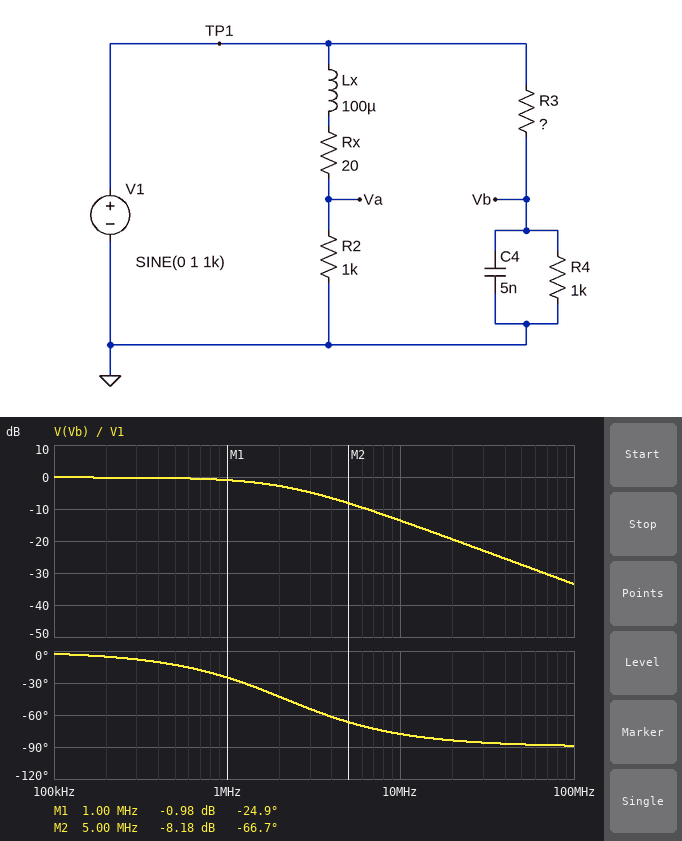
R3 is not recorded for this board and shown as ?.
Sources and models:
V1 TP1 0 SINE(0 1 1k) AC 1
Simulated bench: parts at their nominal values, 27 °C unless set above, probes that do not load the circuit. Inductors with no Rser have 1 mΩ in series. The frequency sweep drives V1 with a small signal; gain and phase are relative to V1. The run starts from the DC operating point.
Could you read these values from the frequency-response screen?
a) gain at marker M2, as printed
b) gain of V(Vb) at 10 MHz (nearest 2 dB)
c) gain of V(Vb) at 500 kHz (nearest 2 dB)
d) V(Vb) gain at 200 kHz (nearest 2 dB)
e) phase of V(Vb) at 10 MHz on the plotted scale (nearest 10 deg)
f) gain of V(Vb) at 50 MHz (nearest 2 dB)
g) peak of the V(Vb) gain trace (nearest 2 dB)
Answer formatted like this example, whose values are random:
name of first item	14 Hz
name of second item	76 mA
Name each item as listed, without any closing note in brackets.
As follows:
gain at marker M2, as printed	-8.18 dB
gain of V(Vb) at 10 MHz	-14 dB
gain of V(Vb) at 500 kHz	0 dB
V(Vb) gain at 200 kHz	0 dB
phase of V(Vb) at 10 MHz on the plotted scale	-80 deg
gain of V(Vb) at 50 MHz	-28 dB
peak of the V(Vb) gain trace	0 dB
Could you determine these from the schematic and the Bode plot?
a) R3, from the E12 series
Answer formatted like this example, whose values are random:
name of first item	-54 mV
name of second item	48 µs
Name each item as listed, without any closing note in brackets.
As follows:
R3, from the E12 series	15 Ω
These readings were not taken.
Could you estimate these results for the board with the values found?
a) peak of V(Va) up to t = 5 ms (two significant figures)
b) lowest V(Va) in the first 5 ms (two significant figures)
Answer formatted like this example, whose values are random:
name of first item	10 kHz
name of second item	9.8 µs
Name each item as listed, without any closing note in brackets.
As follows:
peak of V(Va) up to t = 5 ms	980 mV
lowest V(Va) in the first 5 ms	-980 mV
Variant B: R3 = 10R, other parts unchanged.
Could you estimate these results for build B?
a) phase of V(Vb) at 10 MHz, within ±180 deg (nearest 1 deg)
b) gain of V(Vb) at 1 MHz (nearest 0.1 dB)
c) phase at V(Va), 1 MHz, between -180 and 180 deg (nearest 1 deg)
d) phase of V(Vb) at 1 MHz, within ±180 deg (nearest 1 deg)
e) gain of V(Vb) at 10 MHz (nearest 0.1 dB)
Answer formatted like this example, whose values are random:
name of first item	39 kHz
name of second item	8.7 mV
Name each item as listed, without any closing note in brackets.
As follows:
phase of V(Vb) at 10 MHz, within ±180 deg	-72 deg
gain of V(Vb) at 1 MHz	-0.5 dB
phase at V(Va), 1 MHz, between -180 and 180 deg	-32 deg
phase of V(Vb) at 1 MHz, within ±180 deg	-17 deg
gain of V(Vb) at 10 MHz	-10.4 dB
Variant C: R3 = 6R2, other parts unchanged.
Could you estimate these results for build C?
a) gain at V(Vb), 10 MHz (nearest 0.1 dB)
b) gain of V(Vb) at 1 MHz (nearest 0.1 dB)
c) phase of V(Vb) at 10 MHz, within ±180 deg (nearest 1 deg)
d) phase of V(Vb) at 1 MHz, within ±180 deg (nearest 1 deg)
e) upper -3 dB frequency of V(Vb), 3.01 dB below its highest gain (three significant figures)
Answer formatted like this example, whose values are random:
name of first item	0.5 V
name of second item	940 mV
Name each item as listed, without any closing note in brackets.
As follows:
gain at V(Vb), 10 MHz	-6.8 dB
gain of V(Vb) at 1 MHz	-0.2 dB
phase of V(Vb) at 10 MHz, within ±180 deg	-63 deg
phase of V(Vb) at 1 MHz, within ±180 deg	-11 deg
upper -3 dB frequency of V(Vb), 3.01 dB below its highest gain	5.17 MHz
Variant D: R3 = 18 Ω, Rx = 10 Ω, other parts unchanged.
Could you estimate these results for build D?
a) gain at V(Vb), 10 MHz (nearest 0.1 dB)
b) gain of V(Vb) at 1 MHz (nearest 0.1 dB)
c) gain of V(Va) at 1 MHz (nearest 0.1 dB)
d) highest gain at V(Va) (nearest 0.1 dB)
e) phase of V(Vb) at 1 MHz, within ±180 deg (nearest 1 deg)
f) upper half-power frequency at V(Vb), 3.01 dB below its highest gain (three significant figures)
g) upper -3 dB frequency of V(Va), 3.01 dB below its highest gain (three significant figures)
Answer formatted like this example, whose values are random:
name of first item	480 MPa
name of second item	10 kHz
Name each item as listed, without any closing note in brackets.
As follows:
gain at V(Vb), 10 MHz	-15.2 dB
gain of V(Vb) at 1 MHz	-1.3 dB
gain of V(Va) at 1 MHz	-1.5 dB
highest gain at V(Va)	-0.1 dB
phase of V(Vb) at 1 MHz, within ±180 deg	-29 deg
upper half-power frequency at V(Vb), 3.01 dB below its highest gain	1.80 MHz
upper -3 dB frequency of V(Va), 3.01 dB below its highest gain	1.61 MHz
